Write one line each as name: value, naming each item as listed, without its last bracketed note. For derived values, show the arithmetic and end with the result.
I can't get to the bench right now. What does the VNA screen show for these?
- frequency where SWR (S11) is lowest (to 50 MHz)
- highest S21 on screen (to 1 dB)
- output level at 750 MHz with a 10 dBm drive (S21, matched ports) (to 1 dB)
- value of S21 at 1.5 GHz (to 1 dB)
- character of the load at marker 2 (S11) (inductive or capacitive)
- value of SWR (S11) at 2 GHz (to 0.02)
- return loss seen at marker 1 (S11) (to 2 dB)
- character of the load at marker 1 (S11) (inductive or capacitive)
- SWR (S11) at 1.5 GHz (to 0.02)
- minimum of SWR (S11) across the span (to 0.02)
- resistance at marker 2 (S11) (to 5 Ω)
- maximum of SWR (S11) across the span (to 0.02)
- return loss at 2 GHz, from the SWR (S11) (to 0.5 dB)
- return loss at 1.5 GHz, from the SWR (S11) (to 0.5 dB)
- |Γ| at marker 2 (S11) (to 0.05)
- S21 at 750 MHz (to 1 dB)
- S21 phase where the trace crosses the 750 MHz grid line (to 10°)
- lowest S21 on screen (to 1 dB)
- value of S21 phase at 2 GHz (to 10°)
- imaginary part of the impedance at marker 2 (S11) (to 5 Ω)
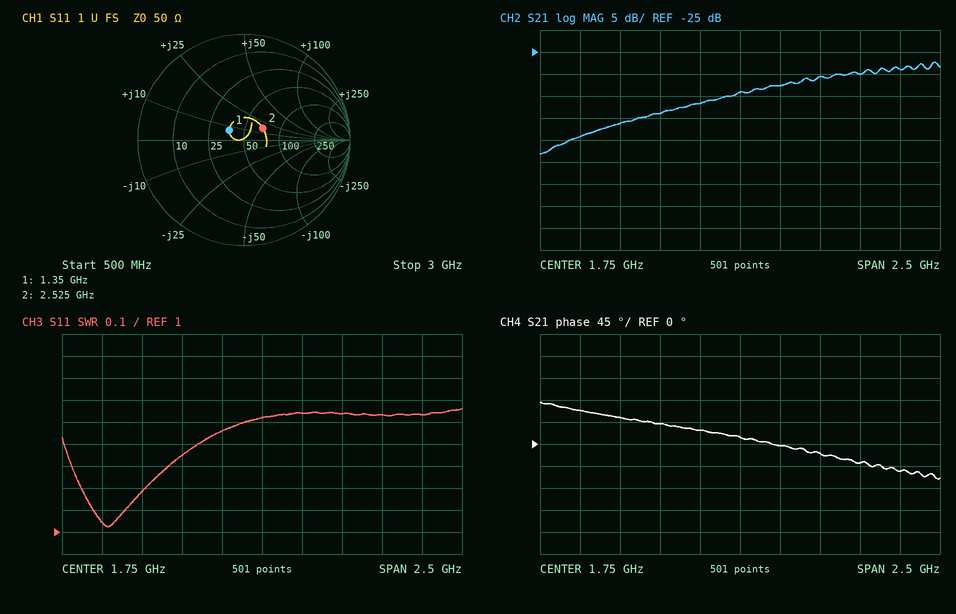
frequency where SWR (S11) is lowest: 800 MHz
highest S21 on screen: -27 dB
output level at 750 MHz with a 10 dBm drive (S21, matched ports): 10 dBm + (-44 dB) = -34 dBm
value of S21 at 1.5 GHz: -37 dB
character of the load at marker 2 (S11): inductive
value of SWR (S11) at 2 GHz: 1.54
return loss seen at marker 1 (S11): 16 dB
character of the load at marker 1 (S11): inductive
SWR (S11) at 1.5 GHz: 1.46
minimum of SWR (S11) across the span: 1.02
resistance at marker 2 (S11): 70 Ω
maximum of SWR (S11) across the span: 1.56
return loss at 2 GHz, from the SWR (S11): −20 log10((1.54 − 1)/(1.54 + 1)) ≈ 13.4 dB, so 13.5 dB to the nearest 0.5 dB
return loss at 1.5 GHz, from the SWR (S11): −20 log10((1.46 − 1)/(1.46 + 1)) ≈ 14.6 dB, so 14.5 dB to the nearest 0.5 dB
|Γ| at marker 2 (S11): 0.20
S21 at 750 MHz: -44 dB
S21 phase where the trace crosses the 750 MHz grid line: 70°
lowest S21 on screen: -48 dB
value of S21 phase at 2 GHz: 0°
imaginary part of the impedance at marker 2 (S11): +15 Ω
